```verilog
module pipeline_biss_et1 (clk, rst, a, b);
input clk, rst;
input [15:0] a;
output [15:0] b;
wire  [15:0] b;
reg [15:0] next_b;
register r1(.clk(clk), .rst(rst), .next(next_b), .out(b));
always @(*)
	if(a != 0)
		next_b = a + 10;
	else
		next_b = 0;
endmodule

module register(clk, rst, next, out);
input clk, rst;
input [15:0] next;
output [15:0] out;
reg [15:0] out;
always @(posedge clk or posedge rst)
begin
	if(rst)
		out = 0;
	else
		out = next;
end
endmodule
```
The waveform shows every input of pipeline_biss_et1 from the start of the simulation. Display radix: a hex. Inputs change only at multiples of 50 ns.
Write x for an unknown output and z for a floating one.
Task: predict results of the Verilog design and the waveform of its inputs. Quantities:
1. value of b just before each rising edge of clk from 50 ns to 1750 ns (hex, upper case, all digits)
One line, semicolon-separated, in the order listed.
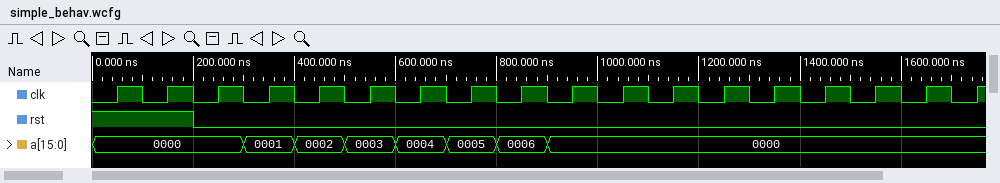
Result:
0000, 0000, 0000, 0000, 000B, 000C, 000D, 000E, 000F, 0010, 0000, 0000, 0000, 0000, 0000, 0000, 0000, 0000
